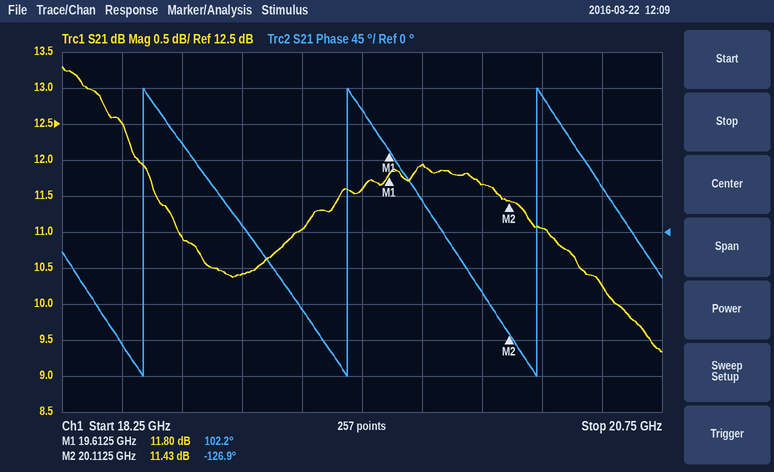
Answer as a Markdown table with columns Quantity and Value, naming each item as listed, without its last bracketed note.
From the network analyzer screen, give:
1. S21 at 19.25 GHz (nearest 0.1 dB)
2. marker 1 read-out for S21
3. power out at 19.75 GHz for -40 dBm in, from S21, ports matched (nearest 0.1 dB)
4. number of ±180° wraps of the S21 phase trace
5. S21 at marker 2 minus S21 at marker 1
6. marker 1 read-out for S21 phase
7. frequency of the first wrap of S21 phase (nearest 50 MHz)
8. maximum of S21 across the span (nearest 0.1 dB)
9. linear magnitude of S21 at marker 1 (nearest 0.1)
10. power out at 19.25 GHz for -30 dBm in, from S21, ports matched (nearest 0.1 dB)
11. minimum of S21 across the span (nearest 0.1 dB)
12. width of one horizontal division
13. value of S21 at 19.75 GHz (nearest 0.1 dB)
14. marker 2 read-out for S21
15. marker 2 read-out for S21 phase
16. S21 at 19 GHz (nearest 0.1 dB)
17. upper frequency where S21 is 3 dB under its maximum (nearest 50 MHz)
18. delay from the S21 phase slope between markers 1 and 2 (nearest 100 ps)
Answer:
| Quantity | Value |
|---|---|
| S21 at 19.25 GHz | 11.0 dB |
| marker 1 read-out for S21 | 11.80 dB |
| power out at 19.75 GHz for -40 dBm in, from S21, ports matched | -28.1 dBm |
| number of ±180° wraps of the S21 phase trace | 3 |
| S21 at marker 2 minus S21 at marker 1 | -0.37 dB |
| marker 1 read-out for S21 phase | 102.2° |
| frequency of the first wrap of S21 phase | 18.60 GHz |
| maximum of S21 across the span | 13.3 dB |
| linear magnitude of S21 at marker 1 | 3.9 |
| power out at 19.25 GHz for -30 dBm in, from S21, ports matched | -19.0 dBm |
| minimum of S21 across the span | 9.3 dB |
| width of one horizontal division | 250 MHz |
| value of S21 at 19.75 GHz | 11.9 dB |
| marker 2 read-out for S21 | 11.43 dB |
| marker 2 read-out for S21 phase | -126.9° |
| S21 at 19 GHz | 10.4 dB |
| upper frequency where S21 is 3 dB under its maximum | 20.50 GHz |
| delay from the S21 phase slope between markers 1 and 2 | 1.3 ns |
